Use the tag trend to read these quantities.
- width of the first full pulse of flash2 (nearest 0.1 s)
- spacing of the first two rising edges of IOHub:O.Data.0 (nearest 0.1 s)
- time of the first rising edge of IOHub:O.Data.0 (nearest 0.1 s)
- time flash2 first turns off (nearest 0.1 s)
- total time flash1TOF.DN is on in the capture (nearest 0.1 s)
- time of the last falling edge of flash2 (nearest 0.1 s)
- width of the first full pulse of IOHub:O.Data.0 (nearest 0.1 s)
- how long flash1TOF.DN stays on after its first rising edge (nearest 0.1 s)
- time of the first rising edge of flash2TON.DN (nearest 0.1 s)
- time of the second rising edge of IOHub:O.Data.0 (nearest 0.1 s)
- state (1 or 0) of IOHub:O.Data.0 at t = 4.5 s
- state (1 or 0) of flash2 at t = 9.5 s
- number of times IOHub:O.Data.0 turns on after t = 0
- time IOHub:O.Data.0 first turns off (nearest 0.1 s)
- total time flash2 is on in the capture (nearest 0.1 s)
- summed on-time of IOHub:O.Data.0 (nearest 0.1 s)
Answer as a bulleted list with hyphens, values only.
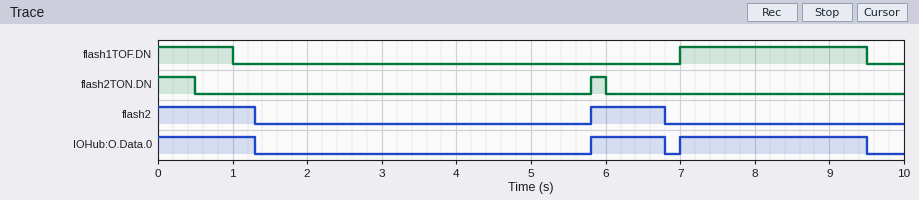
- 1.0 s
- 1.2 s
- 5.8 s
- 1.3 s
- 3.5 s
- 6.8 s
- 1.0 s
- 2.5 s
- 5.8 s
- 7.0 s
- 0
- 0
- 2
- 1.3 s
- 2.3 s
- 4.8 s
